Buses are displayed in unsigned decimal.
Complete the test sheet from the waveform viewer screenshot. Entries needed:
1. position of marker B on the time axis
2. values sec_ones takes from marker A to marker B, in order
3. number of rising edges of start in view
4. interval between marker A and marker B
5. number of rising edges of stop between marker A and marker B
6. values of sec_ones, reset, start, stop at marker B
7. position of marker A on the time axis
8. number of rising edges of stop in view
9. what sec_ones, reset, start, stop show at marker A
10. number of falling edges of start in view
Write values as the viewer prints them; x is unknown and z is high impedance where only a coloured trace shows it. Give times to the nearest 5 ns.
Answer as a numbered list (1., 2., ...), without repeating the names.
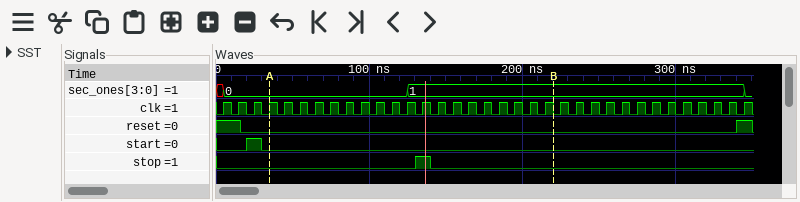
1. 220 ns
2. 0, 1
3. 1
4. 185 ns
5. 1
6. sec_ones=1, reset=0, start=0, stop=0
7. 35 ns
8. 1
9. sec_ones=0, reset=0, start=0, stop=0
10. 1
